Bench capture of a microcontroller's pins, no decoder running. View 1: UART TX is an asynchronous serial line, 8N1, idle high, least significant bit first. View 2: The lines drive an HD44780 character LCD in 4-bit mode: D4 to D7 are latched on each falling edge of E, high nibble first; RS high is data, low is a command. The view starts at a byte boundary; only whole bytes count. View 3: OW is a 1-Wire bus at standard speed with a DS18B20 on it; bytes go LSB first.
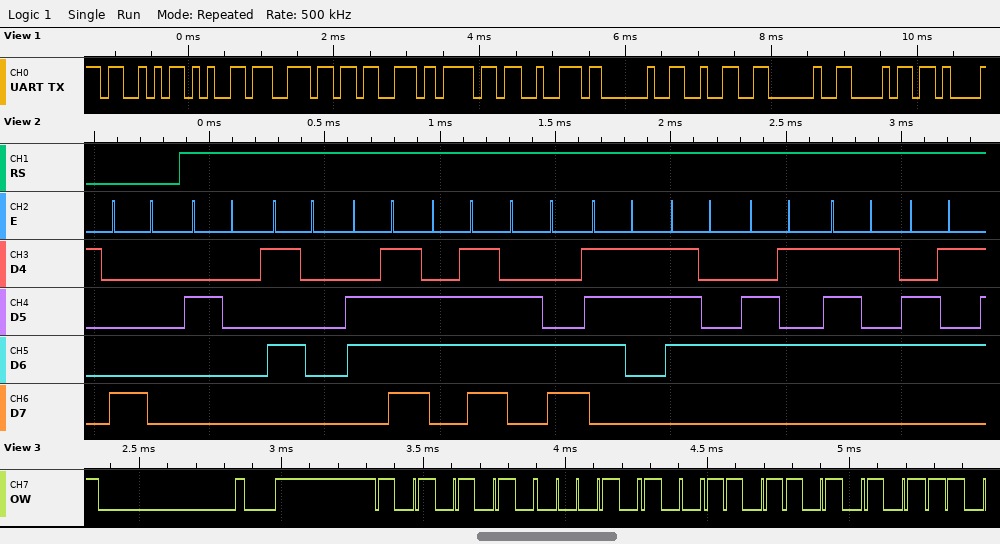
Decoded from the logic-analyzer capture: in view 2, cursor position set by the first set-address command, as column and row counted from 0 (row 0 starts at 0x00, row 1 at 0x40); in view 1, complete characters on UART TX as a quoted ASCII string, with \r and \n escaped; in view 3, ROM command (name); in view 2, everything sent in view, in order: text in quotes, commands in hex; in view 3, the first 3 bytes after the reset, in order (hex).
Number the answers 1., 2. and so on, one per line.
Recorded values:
1. column 0, row 0
2. "Sensor 2 h"
3. Match ROM
4. 0x80 " Poolsteue"
5. 55 28 5B
